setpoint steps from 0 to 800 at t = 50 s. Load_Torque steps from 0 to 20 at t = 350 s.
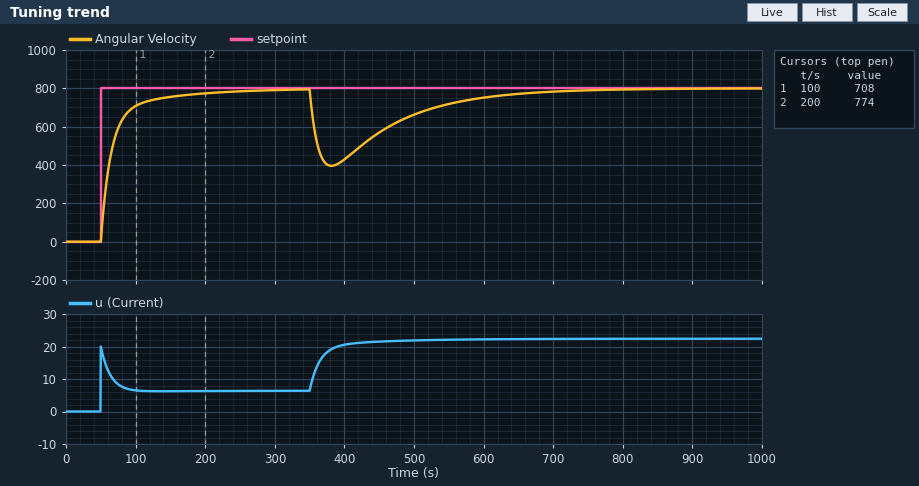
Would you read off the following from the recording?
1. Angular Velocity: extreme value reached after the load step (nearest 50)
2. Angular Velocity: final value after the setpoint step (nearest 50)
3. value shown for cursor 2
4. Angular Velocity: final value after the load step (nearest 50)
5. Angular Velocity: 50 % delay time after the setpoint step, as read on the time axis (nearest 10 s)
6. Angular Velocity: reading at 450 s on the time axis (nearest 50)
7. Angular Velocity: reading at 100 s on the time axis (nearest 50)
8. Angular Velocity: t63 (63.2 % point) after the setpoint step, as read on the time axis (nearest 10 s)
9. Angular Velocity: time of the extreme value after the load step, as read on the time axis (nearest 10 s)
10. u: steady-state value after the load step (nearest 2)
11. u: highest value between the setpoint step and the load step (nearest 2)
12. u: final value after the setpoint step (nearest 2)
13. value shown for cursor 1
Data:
400
800
774
800
60 s
550
700
70 s
380 s
22
20
6
708
